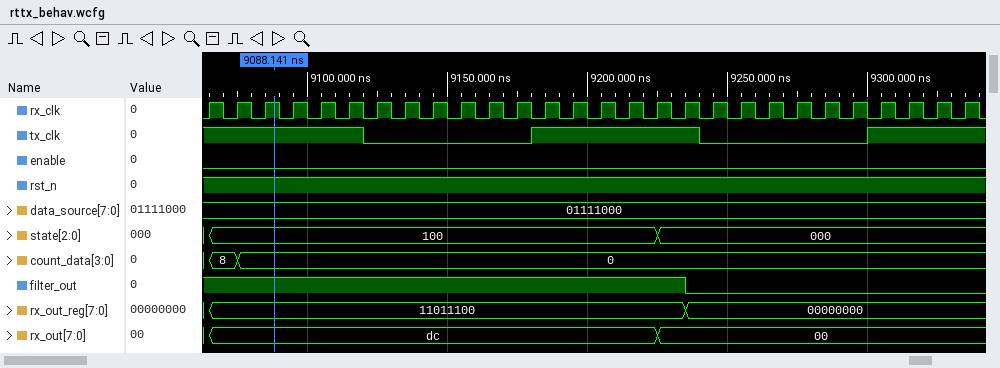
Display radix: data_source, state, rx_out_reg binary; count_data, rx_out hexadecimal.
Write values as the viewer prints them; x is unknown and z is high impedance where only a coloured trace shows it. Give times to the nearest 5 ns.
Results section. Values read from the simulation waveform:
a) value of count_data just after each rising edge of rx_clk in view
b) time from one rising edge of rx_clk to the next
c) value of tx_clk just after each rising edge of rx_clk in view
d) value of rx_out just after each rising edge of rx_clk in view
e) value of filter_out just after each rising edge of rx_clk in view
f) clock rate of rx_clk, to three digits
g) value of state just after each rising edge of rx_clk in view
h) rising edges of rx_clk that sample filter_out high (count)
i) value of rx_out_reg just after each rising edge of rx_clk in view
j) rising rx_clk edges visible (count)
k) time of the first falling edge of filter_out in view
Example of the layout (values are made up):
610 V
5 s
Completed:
8, 0, 0, 0, 0, 0, 0, 0, 0, 0, 0, 0, 0, 0, 0, 0, 0, 0, 0, 0, 0, 0, 0, 0, 0, 0, 0, 0
10 ns
1 1 1 1 1 1 0 0 0 0 0 0 1 1 1 1 1 1 0 0 0 0 0 0 1 1 1 1
dc, dc, dc, dc, dc, dc, dc, dc, dc, dc, dc, dc, dc, dc, dc, dc, 00, 00, 00, 00, 00, 00, 00, 00, 00, 00, 00, 00
1 1 1 1 1 1 1 1 1 1 1 1 1 1 1 1 1 0 0 0 0 0 0 0 0 0 0 0
100 MHz
100, 100, 100, 100, 100, 100, 100, 100, 100, 100, 100, 100, 100, 100, 100, 100, 000, 000, 000, 000, 000, 000, 000, 000, 000, 000, 000, 000
18
11011100, 11011100, 11011100, 11011100, 11011100, 11011100, 11011100, 11011100, 11011100, 11011100, 11011100, 11011100, 11011100, 11011100, 11011100, 11011100, 11011100, 00000000, 00000000, 00000000, 00000000, 00000000, 00000000, 00000000, 00000000, 00000000, 00000000, 00000000
28
9235 ns
